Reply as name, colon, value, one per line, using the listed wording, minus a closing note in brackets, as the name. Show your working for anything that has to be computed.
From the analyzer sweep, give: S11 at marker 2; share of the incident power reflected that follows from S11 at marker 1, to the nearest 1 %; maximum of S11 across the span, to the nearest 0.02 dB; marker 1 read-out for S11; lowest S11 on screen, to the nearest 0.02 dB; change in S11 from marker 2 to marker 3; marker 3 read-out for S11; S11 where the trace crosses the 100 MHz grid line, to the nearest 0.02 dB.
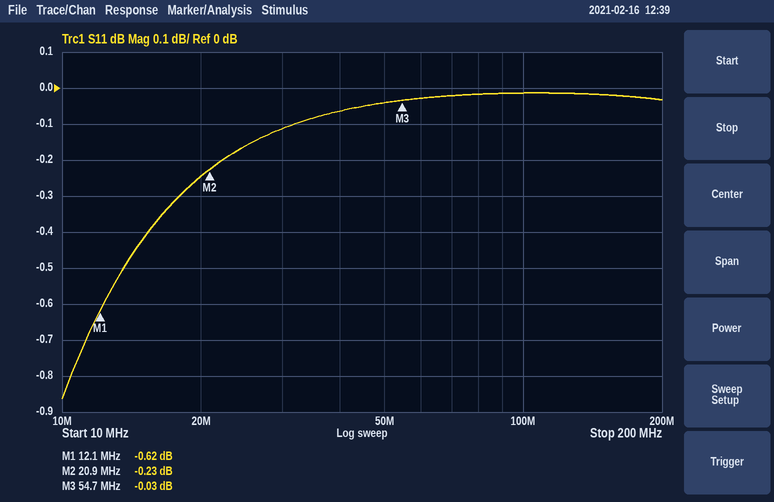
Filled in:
S11 at marker 2: -0.23 dB
share of the incident power reflected that follows from S11 at marker 1, to the nearest 1 %: 10^(-0.62/10) ≈ 87 %
maximum of S11 across the span, to the nearest 0.02 dB: -0.02 dB
marker 1 read-out for S11: -0.62 dB
lowest S11 on screen, to the nearest 0.02 dB: -0.86 dB
change in S11 from marker 2 to marker 3: -0.03 − (-0.23) = 0.20 dB
marker 3 read-out for S11: -0.03 dB
S11 where the trace crosses the 100 MHz grid line, to the nearest 0.02 dB: -0.02 dB
